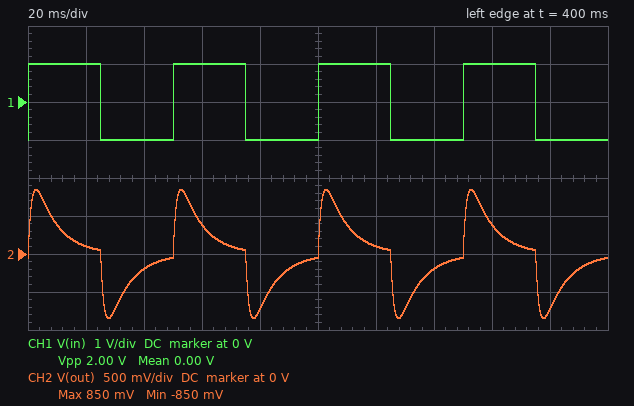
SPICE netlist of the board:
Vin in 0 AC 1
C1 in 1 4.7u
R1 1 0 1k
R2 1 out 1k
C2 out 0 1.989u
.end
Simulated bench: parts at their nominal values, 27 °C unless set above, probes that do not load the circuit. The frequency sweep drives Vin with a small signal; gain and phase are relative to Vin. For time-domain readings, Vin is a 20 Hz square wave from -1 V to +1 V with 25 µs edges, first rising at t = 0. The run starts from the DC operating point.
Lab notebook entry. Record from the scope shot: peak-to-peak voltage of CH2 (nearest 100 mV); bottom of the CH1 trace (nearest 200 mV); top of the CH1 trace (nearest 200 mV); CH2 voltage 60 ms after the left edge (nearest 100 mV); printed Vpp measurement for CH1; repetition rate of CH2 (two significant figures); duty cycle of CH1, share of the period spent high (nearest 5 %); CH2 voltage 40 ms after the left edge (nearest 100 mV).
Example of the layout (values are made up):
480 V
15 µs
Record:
1.7 V
-1.0 V
1.0 V
400 mV
2.00 V
20 Hz
50 %
-200 mV
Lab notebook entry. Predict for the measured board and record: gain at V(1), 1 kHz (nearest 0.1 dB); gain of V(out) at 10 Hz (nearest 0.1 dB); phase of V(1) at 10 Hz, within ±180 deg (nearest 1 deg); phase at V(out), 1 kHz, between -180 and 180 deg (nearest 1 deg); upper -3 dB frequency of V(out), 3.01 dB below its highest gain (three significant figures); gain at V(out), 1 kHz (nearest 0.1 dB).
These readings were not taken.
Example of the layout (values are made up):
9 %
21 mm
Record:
0 dB
-11.5 dB
68 deg
-82 deg
164 Hz
-22.0 dB
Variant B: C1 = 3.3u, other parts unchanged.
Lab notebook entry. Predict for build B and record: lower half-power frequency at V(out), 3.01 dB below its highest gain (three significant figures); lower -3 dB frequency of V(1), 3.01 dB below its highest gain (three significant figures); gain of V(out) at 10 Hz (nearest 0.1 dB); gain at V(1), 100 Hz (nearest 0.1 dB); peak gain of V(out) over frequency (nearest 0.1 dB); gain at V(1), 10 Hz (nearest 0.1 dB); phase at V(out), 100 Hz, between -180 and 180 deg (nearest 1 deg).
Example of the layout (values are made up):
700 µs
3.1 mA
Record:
19.7 Hz
109 Hz
-14.3 dB
-3.3 dB
-6.9 dB
-14.2 dB
-19 deg
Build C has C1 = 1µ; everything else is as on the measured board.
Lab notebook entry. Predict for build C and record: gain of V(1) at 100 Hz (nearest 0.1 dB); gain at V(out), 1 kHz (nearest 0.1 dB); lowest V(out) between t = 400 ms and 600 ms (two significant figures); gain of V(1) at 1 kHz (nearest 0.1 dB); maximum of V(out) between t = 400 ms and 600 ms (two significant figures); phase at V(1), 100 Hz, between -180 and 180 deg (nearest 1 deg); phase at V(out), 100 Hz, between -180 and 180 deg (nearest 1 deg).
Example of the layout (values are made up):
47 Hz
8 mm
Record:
-9.9 dB
-22.5 dB
-340 mV
-0.5 dB
340 mV
55 deg
4 deg
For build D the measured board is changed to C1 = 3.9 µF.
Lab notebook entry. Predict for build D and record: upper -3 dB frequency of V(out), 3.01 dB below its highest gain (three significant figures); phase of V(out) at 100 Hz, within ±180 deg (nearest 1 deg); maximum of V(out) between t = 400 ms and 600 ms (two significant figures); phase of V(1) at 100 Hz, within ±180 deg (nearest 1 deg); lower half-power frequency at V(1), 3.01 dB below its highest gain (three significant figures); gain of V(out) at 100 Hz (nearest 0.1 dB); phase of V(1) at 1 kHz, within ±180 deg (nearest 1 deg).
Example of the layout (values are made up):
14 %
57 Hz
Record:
180 Hz
-23 deg
780 mV
29 deg
90.0 Hz
-6.8 dB
5 deg
